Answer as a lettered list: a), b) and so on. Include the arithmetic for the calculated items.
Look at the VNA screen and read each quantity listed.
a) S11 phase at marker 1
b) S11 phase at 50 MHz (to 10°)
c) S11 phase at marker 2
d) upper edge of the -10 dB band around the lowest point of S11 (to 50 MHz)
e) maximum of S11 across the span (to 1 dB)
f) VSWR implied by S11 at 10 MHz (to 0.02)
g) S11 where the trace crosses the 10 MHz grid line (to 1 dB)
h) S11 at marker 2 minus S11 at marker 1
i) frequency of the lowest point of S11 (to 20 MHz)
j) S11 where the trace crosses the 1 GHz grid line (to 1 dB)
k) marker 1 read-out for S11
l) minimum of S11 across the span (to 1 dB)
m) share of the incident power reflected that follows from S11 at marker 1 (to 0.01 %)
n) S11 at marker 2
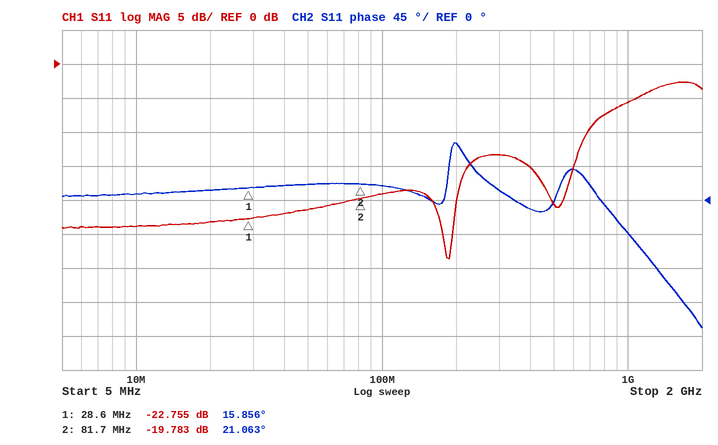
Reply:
a) 15.856°
b) 20°
c) 21.063°
d) 700 MHz
e) -3 dB
f) |Γ| = 10^(-24/20) = 0.0631; VSWR = (1 + 0.0631)/(1 − 0.0631) ≈ 1.13, so 1.14 to the nearest 0.02
g) -24 dB
h) -19.783 − (-22.755) = 2.972 dB
i) 180 MHz
j) -6 dB
k) -22.755 dB
l) -29 dB
m) 10^(-22.755/10) ≈ 0.53 %
n) -19.783 dB
